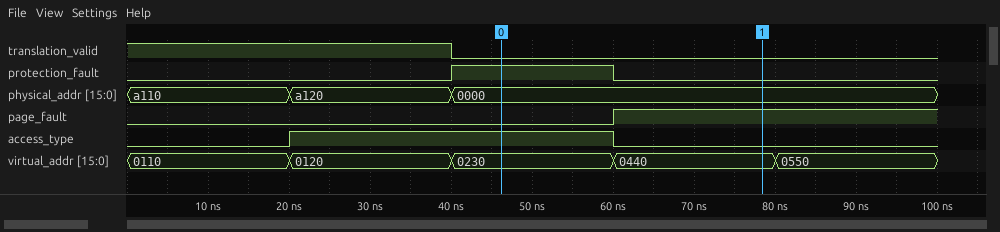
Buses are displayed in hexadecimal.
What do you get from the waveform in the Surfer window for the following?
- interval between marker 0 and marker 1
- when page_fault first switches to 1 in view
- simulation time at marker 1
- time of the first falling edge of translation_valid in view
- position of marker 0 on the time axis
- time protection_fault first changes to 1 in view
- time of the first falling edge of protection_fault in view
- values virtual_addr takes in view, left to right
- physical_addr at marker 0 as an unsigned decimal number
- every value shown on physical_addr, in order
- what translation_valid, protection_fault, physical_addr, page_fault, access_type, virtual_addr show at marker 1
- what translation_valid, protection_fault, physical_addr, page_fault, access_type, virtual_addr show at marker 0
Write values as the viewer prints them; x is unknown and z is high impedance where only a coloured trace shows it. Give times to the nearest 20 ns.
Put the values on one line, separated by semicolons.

40 ns; 60 ns; 80 ns; 40 ns; 40 ns; 40 ns; 60 ns; 0110, 0120, 0230, 0440, 0550; 0; a110, a120, 0000; translation_valid=0, protection_fault=0, physical_addr=0000, page_fault=1, access_type=0, virtual_addr=0440; translation_valid=0, protection_fault=1, physical_addr=0000, page_fault=0, access_type=1, virtual_addr=0230
